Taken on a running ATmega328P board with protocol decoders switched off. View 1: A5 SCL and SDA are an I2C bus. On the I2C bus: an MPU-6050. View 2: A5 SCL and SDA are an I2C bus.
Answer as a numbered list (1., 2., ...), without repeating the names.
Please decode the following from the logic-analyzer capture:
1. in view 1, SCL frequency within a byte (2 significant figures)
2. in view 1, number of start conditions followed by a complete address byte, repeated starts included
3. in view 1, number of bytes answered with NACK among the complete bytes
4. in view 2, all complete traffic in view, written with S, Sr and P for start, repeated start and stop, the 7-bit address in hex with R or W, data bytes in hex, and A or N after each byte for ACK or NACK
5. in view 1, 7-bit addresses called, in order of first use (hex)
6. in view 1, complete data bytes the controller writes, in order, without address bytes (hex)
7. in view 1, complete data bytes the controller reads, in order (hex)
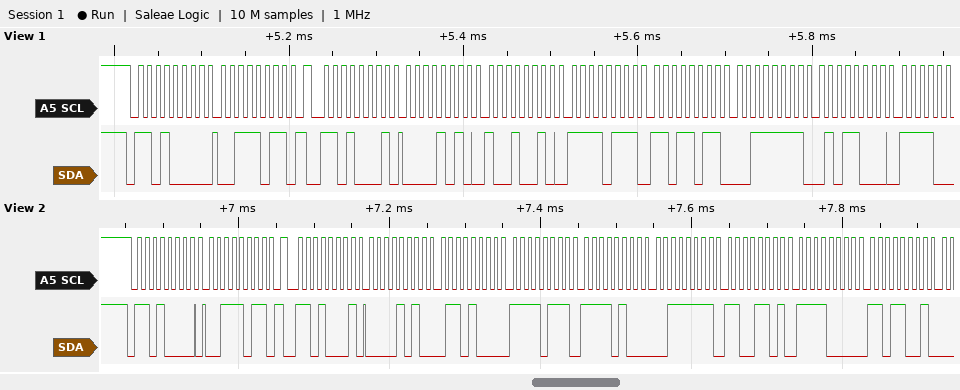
1. 100 kHz
2. 2
3. 0
4. S 68W A 3B A Sr 68R A 0A A 68 A F7 A F4 A 3F A CD A F0 A D9 A
5. 0x68
6. 3B
7. 0A 92 F7 DB 3F 58
